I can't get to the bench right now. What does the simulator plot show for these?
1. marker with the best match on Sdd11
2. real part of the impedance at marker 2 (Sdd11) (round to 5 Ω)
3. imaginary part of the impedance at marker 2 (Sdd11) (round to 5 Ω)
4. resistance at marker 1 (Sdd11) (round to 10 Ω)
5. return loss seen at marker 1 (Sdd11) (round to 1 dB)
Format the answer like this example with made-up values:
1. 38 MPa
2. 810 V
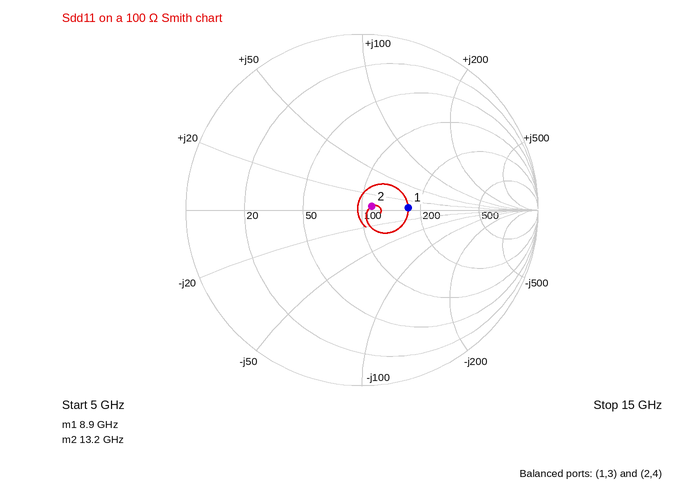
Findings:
1. marker 2
2. 110 Ω
3. +5 Ω
4. 170 Ω
5. 12 dB
